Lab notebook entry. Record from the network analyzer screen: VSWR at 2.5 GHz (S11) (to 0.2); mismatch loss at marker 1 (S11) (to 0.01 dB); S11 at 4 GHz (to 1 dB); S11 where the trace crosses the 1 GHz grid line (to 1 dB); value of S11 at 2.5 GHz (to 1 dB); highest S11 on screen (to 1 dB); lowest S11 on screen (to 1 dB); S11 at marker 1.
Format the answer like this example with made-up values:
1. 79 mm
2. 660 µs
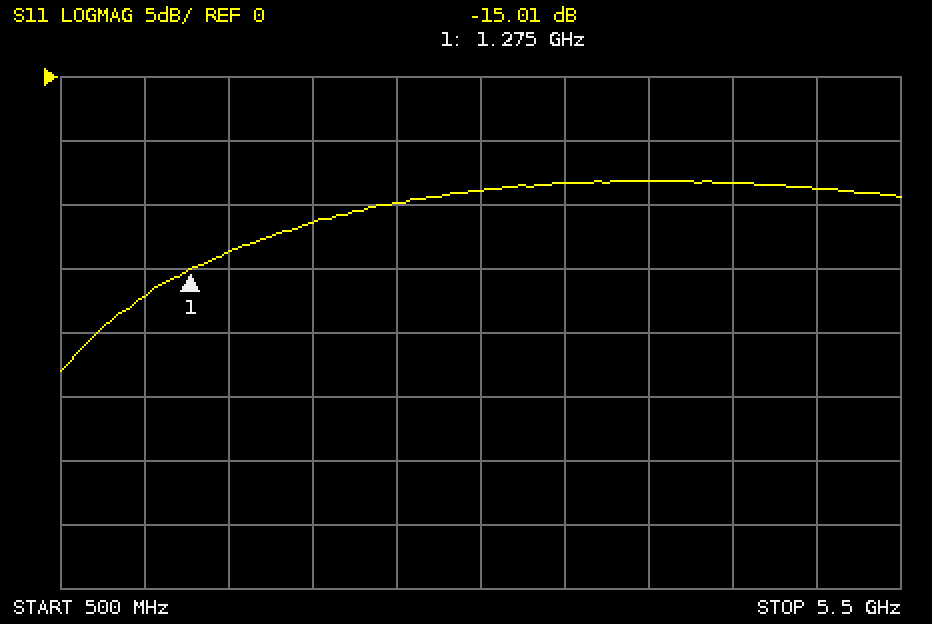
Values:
1. 2.0
2. 0.14 dB
3. -8 dB
4. -17 dB
5. -10 dB
6. -8 dB
7. -23 dB
8. -15.01 dB
